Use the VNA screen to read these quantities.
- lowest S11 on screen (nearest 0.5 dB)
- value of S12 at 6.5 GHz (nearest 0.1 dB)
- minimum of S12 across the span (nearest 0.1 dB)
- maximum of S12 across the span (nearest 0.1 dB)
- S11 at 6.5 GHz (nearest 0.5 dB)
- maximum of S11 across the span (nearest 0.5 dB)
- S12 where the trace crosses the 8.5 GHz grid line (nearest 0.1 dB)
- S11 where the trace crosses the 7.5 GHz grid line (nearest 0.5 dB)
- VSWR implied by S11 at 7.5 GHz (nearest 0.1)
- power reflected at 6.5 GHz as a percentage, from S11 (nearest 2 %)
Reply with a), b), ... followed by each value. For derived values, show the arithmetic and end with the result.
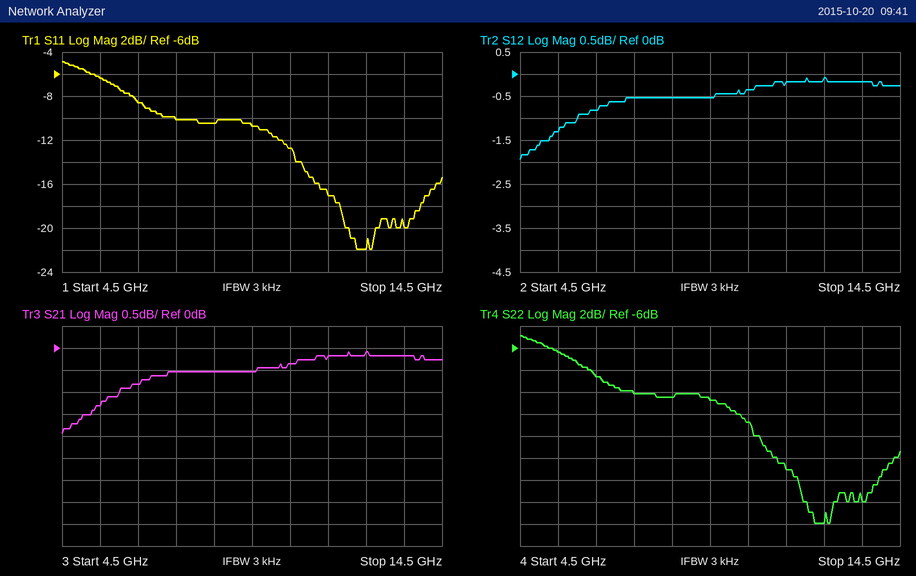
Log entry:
a) -22.0 dB
b) -0.8 dB
c) -1.9 dB
d) -0.1 dB
e) -8.5 dB
f) -5.0 dB
g) -0.5 dB
h) -10.0 dB
i) |Γ| = 10^(-10/20) = 0.3162; VSWR = (1 + 0.3162)/(1 − 0.3162) ≈ 1.9
j) 10^(-8.5/10) ≈ 14 %
